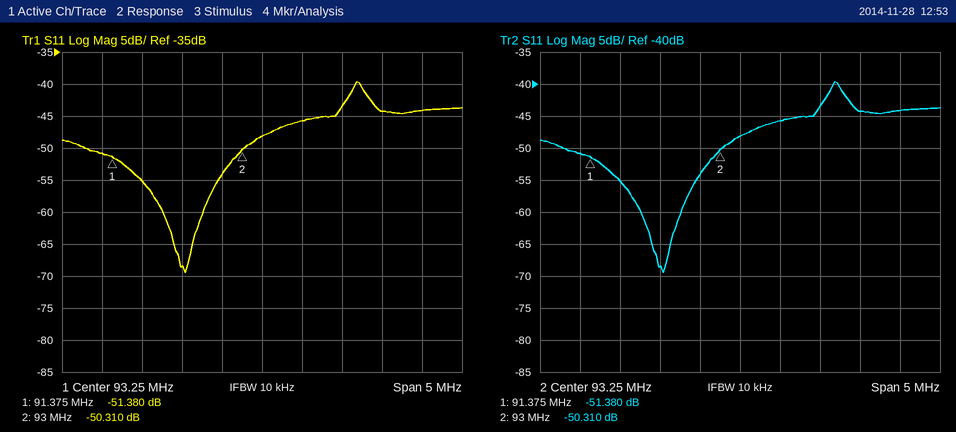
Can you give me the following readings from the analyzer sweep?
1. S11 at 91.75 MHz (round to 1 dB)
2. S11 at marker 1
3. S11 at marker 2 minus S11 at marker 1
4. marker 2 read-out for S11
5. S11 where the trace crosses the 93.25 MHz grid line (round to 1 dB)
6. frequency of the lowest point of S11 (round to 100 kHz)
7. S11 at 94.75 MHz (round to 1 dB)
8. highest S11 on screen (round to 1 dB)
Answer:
-55 dB
-51.380 dB
1.070 dB
-50.310 dB
-48 dB
92.3 MHz
-44 dB
-40 dB
